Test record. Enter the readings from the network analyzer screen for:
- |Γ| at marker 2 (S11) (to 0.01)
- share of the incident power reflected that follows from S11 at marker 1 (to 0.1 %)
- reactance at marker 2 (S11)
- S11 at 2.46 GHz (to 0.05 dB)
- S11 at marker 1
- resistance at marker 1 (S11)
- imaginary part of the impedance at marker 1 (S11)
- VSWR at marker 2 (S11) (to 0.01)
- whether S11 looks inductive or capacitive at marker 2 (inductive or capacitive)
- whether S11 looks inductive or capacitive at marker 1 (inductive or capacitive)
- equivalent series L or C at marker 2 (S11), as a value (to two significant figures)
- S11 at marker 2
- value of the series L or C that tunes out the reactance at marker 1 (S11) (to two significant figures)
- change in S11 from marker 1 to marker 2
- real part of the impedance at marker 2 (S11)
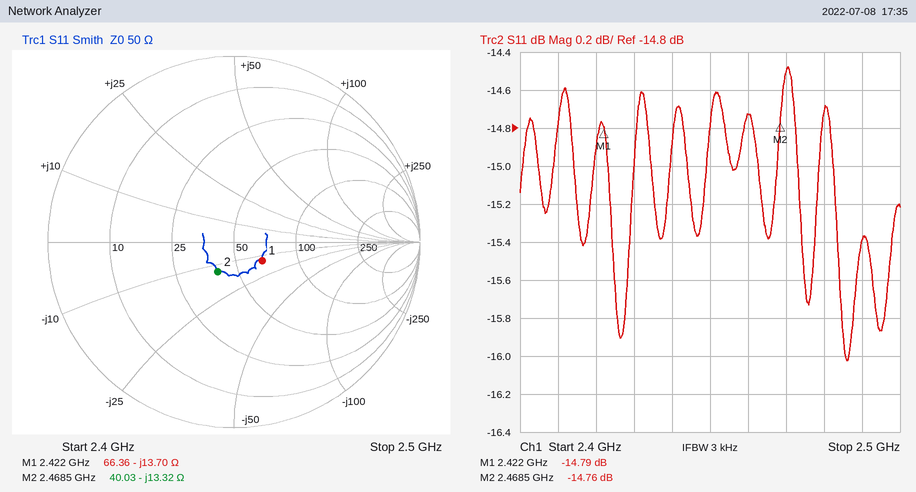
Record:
0.18
3.3 %
-13.32 Ω
-14.75 dB
-14.79 dB
66.36 Ω
-13.70 Ω
1.45
capacitive
capacitive
4.8 pF
-14.76 dB
900 pH
0.03 dB
40.03 Ω
